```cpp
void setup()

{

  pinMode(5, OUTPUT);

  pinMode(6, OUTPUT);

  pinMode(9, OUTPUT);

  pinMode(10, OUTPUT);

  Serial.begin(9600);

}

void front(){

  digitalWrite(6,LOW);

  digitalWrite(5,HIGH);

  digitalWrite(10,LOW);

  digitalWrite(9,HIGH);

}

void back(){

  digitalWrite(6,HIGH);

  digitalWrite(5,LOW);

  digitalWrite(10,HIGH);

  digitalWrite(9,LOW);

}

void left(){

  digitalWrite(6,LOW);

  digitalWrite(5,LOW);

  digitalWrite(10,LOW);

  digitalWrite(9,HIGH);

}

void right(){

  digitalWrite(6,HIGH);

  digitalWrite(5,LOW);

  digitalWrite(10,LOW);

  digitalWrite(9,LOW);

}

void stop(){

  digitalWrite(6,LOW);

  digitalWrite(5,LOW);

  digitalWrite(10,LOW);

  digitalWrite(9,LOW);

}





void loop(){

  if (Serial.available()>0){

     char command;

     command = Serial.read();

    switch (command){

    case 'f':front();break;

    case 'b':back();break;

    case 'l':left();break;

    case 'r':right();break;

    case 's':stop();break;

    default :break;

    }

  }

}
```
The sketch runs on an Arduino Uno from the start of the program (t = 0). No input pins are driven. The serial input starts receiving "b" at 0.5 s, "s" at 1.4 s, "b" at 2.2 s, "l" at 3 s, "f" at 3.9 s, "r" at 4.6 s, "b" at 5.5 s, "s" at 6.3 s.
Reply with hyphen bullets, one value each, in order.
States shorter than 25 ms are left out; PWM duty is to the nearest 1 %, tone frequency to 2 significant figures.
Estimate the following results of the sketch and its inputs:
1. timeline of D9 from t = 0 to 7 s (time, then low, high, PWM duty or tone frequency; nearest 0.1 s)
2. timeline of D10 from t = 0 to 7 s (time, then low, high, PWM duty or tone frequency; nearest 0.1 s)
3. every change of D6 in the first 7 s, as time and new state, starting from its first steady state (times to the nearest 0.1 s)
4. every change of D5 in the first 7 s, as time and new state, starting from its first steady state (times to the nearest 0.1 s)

- 0 s low; 3 s high; 4.6 s low
- 0 s low; 0.5 s high; 1.4 s low; 2.2 s high; 3 s low; 5.5 s high; 6.3 s low
- 0 s low; 0.5 s high; 1.4 s low; 2.2 s high; 3 s low; 4.6 s high; 6.3 s low
- 0 s low; 3.9 s high; 4.6 s low
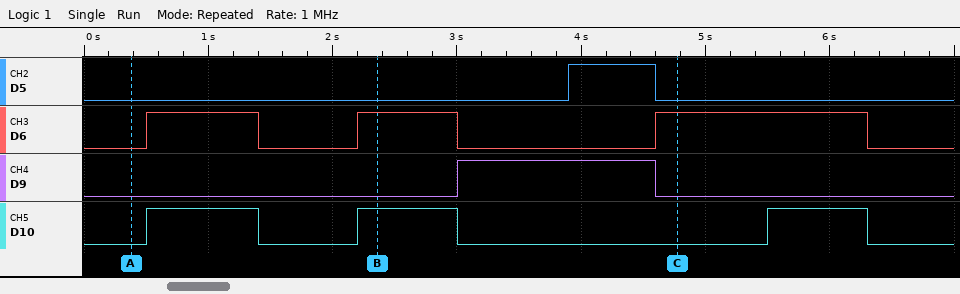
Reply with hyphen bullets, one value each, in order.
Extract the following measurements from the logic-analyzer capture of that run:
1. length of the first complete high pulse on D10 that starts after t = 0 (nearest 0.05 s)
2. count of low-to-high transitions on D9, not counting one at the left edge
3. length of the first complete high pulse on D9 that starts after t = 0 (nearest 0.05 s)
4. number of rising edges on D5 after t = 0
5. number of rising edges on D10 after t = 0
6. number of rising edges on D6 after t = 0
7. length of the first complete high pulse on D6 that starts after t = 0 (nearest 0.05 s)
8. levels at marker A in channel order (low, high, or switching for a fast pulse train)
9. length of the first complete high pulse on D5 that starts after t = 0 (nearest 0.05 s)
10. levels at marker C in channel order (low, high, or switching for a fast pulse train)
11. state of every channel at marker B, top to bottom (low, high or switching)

- 0.90 s
- 1
- 1.60 s
- 1
- 3
- 3
- 0.90 s
- D5 low, D6 low, D9 low, D10 low
- 0.70 s
- D5 low, D6 high, D9 low, D10 low
- D5 low, D6 high, D9 low, D10 high
